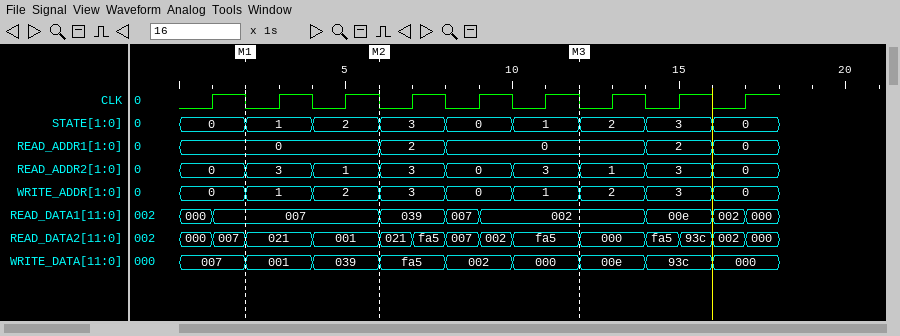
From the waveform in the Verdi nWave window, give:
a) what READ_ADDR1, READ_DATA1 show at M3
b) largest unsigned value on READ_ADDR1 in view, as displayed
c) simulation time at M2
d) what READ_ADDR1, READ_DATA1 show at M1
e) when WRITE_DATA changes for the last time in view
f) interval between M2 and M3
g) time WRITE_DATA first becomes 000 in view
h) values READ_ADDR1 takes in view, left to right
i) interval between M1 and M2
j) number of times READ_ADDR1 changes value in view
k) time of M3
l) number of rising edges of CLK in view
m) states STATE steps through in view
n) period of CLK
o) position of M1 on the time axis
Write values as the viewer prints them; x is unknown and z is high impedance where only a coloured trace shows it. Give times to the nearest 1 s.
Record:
READ_ADDR1=0, READ_DATA1=002
2
6 s
READ_ADDR1=0, READ_DATA1=007
16 s
6 s
10 s
0, 2, 0, 2, 0
4 s
4
12 s
9
0, 1, 2, 3, 0, 1, 2, 3, 0
2 s
2 s
